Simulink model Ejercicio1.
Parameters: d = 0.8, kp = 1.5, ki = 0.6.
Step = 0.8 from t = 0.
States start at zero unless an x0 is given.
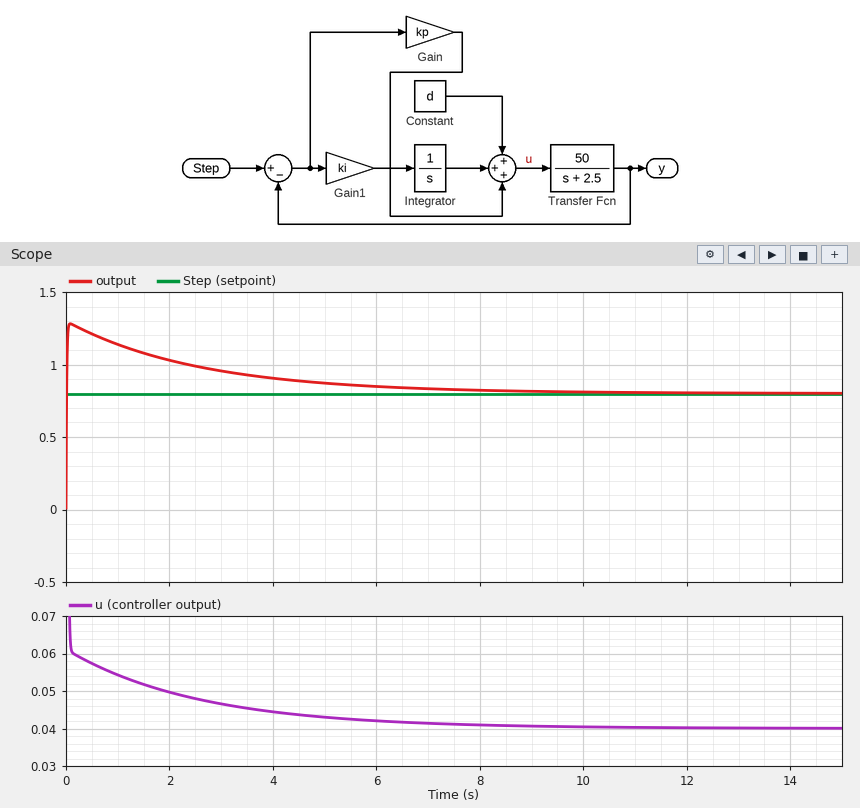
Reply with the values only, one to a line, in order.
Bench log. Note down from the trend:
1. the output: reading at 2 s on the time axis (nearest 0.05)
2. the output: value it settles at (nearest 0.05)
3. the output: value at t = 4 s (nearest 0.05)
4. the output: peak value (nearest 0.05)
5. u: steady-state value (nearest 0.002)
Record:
1.05
0.80
0.90
1.30
0.040
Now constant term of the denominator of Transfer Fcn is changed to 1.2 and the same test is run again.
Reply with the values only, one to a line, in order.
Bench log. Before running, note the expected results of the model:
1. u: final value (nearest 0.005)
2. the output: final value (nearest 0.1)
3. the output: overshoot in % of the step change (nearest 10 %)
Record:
0.020
0.8
60 %
